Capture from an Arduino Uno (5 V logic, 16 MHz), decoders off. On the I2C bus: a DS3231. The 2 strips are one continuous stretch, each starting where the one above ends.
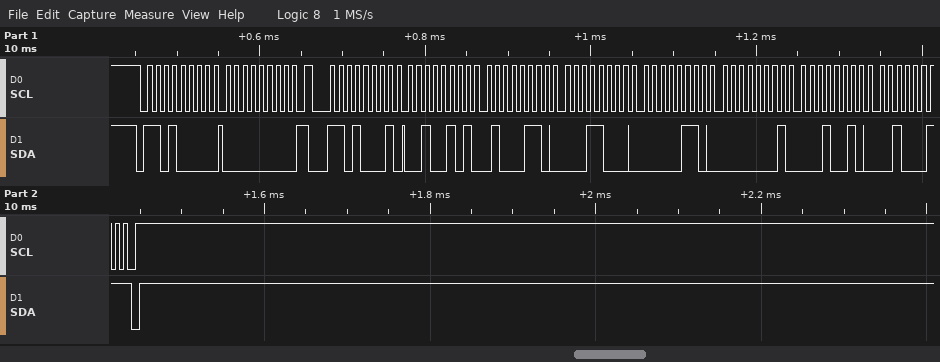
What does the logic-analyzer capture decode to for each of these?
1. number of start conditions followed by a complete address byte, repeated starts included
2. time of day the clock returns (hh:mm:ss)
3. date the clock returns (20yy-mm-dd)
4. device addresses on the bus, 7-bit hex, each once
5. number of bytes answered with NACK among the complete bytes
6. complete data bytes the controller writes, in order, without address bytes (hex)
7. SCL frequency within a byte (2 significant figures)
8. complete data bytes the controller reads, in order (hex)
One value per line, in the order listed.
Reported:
2
18:46:25
2023-12-01
0x68
1
00
100 kHz
25 46 18 06 01 12 23
